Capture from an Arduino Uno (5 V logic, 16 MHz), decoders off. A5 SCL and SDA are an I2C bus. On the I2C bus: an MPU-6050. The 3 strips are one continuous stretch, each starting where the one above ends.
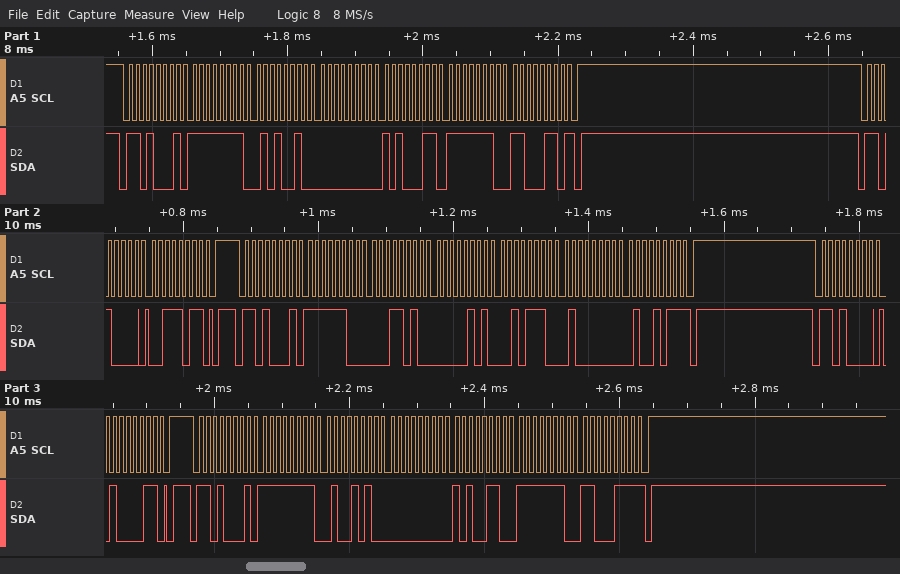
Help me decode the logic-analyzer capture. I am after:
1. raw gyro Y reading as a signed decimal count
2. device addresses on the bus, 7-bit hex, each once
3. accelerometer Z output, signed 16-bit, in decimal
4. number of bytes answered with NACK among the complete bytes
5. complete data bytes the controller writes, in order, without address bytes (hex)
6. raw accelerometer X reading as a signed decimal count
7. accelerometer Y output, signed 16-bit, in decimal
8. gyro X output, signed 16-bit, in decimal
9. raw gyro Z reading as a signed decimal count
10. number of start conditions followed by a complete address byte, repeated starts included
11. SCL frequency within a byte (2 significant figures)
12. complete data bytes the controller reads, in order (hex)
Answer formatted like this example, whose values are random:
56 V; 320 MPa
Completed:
166; 0x68; 16459; 3; 3B 43; -998; 1326; -182; -313; 5; 100 kHz; FF 52 00 A3 FE C6 FC 1A 05 2E 40 4B FF 4A 00 A6 FE C7
